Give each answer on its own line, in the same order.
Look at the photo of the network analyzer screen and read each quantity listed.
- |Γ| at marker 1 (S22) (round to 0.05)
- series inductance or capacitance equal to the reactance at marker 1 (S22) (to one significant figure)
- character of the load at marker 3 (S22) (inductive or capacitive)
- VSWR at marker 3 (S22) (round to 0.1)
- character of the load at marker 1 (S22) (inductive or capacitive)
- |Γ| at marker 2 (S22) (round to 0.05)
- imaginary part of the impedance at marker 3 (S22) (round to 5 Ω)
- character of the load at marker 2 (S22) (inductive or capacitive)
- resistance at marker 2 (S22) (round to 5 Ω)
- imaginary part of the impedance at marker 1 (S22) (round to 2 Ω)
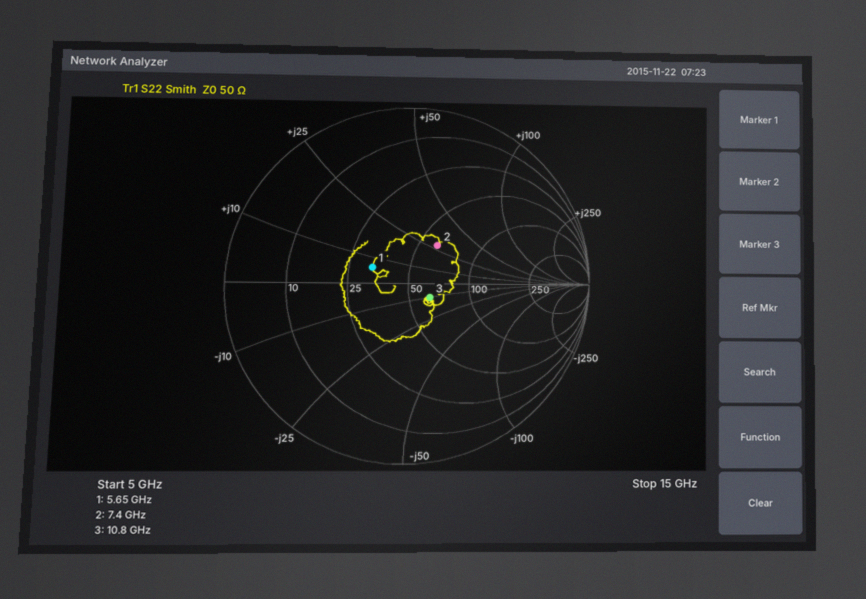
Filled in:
0.20
200 pH
capacitive
1.3
inductive
0.25
-10 Ω
inductive
60 Ω
+6 Ω
